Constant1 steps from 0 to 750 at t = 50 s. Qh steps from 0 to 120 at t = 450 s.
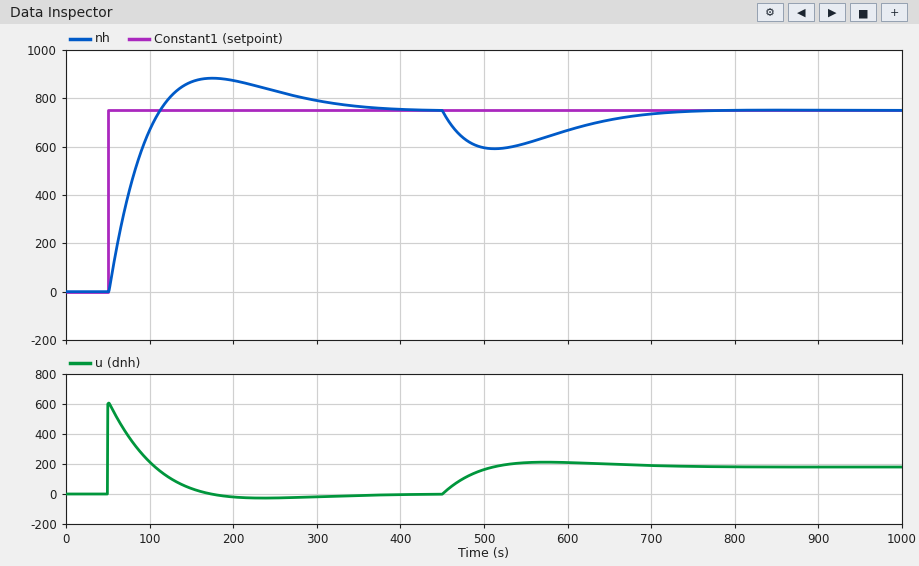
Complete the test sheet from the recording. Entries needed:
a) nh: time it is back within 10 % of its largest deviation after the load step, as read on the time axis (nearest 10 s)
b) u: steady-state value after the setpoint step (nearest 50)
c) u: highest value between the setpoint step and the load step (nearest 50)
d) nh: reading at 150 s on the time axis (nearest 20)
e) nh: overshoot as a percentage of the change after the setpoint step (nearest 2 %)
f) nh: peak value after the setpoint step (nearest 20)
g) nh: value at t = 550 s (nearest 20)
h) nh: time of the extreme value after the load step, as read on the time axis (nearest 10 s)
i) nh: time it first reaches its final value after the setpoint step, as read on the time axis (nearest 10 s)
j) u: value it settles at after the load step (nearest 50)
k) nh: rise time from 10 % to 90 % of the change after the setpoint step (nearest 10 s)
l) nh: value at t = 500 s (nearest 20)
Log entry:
700 s
0
600
860
18 %
880
620
510 s
110 s
200
50 s
600
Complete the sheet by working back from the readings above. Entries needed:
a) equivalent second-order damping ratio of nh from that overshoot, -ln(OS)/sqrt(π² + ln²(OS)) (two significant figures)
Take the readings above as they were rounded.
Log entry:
0.48
